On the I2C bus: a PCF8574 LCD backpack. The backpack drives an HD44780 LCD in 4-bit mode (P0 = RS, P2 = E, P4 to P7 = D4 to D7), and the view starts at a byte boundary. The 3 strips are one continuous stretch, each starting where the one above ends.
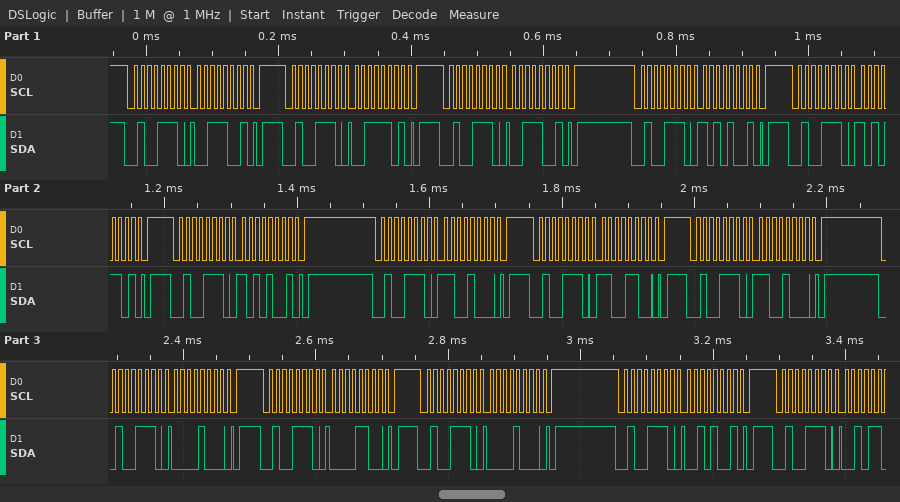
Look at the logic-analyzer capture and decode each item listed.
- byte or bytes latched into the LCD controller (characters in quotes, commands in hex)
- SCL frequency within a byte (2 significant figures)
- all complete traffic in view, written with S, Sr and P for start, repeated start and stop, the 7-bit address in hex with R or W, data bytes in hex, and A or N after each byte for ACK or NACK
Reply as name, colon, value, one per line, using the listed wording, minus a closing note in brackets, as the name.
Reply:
byte or bytes latched into the LCD controller: ':' 0xC0
SCL frequency within a byte: 100 kHz
all complete traffic in view, written with S, Sr and P for start, repeated start and stop, the 7-bit address in hex with R or W, data bytes in hex, and A or N after each byte for ACK or NACK: S 27W A 39 A P S 27W A 3D A P S 27W A 39 A P S 27W A A9 A P S 27W A AD A P S 27W A A9 A P S 27W A C8 A P S 27W A CC A P S 27W A C8 A P S 27W A 08 A P S 27W A 0C A P S 27W A 08 A P S 27W A 29 A P S 27W A
